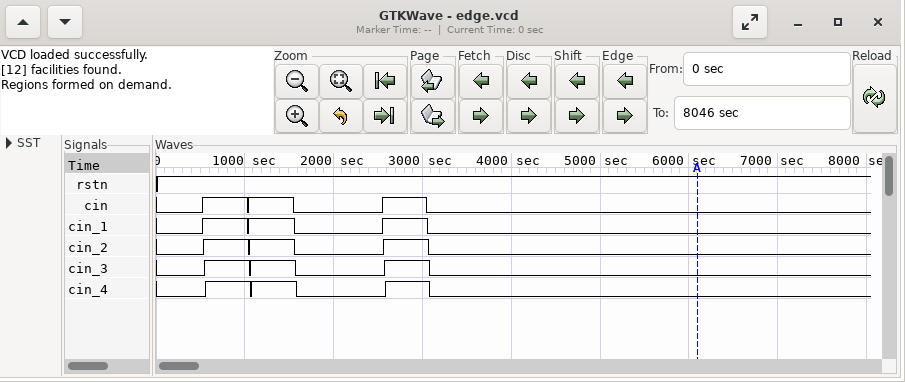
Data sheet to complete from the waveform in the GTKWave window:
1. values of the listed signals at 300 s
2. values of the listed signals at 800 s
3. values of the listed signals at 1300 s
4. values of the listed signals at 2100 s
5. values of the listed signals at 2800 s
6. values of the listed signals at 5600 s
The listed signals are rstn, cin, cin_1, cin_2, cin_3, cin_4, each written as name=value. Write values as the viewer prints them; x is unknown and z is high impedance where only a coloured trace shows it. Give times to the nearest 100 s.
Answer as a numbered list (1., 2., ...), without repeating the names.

1. rstn=1, cin=0, cin_1=0, cin_2=0, cin_3=0, cin_4=0
2. rstn=1, cin=1, cin_1=1, cin_2=1, cin_3=1, cin_4=1
3. rstn=1, cin=1, cin_1=1, cin_2=1, cin_3=1, cin_4=1
4. rstn=1, cin=0, cin_1=0, cin_2=0, cin_3=0, cin_4=0
5. rstn=1, cin=1, cin_1=1, cin_2=1, cin_3=1, cin_4=1
6. rstn=1, cin=0, cin_1=0, cin_2=0, cin_3=0, cin_4=0
